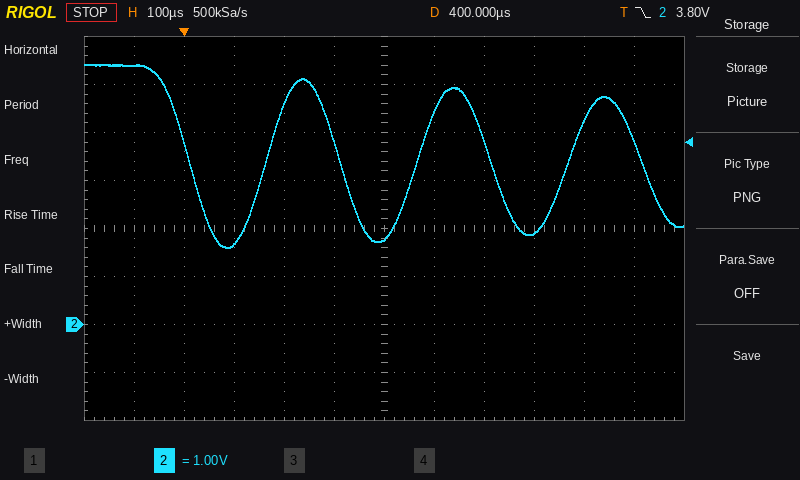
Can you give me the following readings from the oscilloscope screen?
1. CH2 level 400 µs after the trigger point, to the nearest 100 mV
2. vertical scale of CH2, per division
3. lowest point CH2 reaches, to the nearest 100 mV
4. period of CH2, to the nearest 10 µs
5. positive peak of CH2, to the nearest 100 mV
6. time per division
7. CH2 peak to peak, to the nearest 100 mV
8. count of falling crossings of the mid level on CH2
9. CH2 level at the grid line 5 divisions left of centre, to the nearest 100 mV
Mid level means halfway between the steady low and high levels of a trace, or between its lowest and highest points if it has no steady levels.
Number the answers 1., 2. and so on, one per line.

1. 1.8 V
2. 1 V
3. 1.6 V
4. 300 µs
5. 5.4 V
6. 100 µs
7. 3.8 V
8. 4
9. 5.4 V
